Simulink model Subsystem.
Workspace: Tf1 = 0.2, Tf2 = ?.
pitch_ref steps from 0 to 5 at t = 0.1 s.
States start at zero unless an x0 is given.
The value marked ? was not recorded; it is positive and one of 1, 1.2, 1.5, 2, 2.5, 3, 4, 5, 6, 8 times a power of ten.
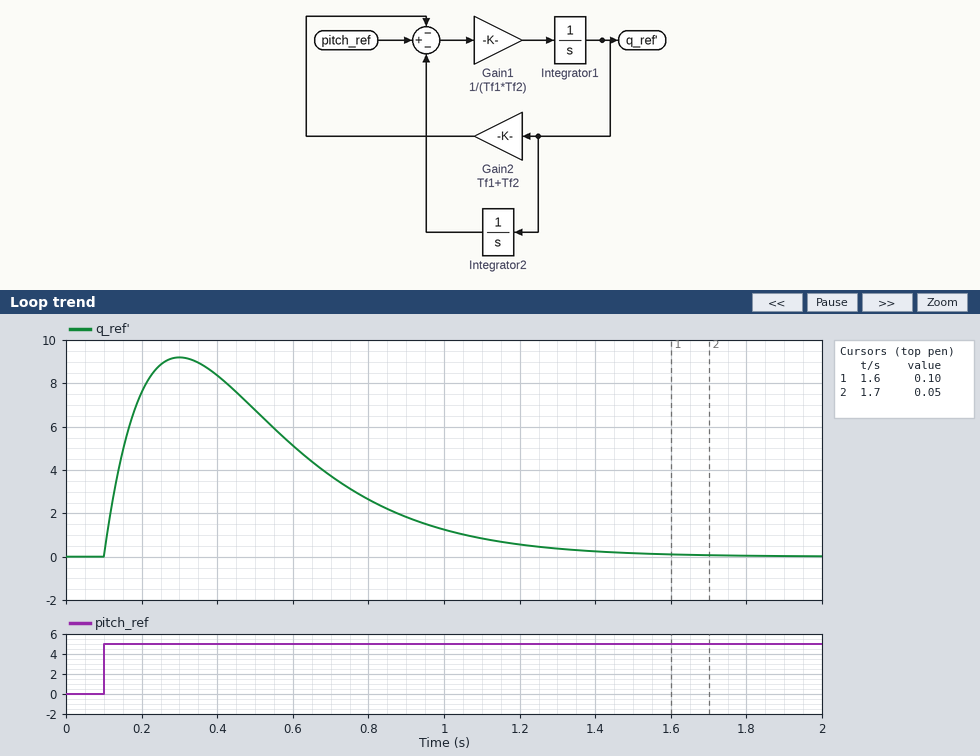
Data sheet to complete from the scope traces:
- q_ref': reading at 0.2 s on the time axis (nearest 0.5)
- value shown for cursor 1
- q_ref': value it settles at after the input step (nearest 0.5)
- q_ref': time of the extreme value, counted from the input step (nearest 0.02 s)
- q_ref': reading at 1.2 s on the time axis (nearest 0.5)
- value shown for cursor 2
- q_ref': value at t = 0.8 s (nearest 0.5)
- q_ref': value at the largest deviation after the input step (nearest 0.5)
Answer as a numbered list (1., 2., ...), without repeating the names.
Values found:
1. 7.5
2. 0.10
3. 0.0
4. 0.20 s
5. 0.5
6. 0.05
7. 2.5
8. 9.0
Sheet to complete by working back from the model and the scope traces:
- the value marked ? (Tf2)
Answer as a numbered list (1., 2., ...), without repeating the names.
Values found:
1. 0.2
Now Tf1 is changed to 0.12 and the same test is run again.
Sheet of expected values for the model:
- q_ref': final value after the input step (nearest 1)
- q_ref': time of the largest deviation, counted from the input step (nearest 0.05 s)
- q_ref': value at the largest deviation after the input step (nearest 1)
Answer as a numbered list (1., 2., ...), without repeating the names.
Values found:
1. 0
2. 0.15 s
3. 12
